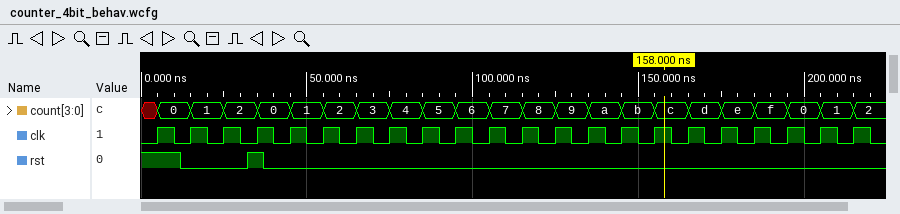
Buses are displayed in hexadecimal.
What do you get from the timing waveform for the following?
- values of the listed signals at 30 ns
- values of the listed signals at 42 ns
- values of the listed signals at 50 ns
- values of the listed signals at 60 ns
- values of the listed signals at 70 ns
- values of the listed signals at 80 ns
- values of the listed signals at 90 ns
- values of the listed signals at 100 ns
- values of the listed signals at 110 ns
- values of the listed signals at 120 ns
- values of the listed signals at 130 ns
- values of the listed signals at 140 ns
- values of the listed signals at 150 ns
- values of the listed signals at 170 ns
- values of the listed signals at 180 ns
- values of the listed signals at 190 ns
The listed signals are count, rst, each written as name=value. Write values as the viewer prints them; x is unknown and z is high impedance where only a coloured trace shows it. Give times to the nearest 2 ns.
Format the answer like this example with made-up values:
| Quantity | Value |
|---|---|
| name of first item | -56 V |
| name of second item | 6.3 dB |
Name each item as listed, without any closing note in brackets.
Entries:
| Quantity | Value |
|---|---|
| values of the listed signals at 30 ns | count=2, rst=0 |
| values of the listed signals at 42 ns | count=0, rst=0 |
| values of the listed signals at 50 ns | count=1, rst=0 |
| values of the listed signals at 60 ns | count=2, rst=0 |
| values of the listed signals at 70 ns | count=3, rst=0 |
| values of the listed signals at 80 ns | count=4, rst=0 |
| values of the listed signals at 90 ns | count=5, rst=0 |
| values of the listed signals at 100 ns | count=6, rst=0 |
| values of the listed signals at 110 ns | count=7, rst=0 |
| values of the listed signals at 120 ns | count=8, rst=0 |
| values of the listed signals at 130 ns | count=9, rst=0 |
| values of the listed signals at 140 ns | count=a, rst=0 |
| values of the listed signals at 150 ns | count=b, rst=0 |
| values of the listed signals at 170 ns | count=d, rst=0 |
| values of the listed signals at 180 ns | count=e, rst=0 |
| values of the listed signals at 190 ns | count=f, rst=0 |
